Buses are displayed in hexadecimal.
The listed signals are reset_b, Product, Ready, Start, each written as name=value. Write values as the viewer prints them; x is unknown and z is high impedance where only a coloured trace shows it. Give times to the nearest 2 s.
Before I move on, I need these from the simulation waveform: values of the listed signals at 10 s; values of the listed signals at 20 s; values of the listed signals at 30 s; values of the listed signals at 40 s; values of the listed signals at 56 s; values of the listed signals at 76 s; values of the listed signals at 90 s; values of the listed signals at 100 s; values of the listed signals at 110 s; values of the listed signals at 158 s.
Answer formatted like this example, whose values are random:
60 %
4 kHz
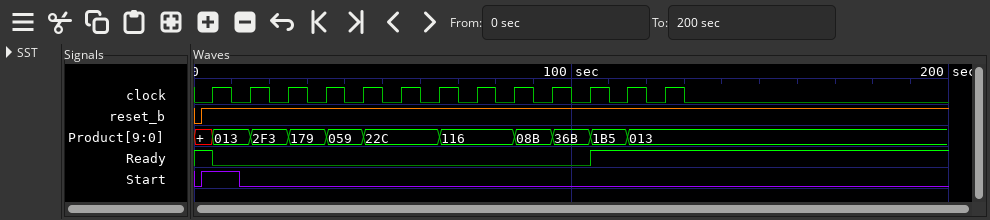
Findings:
reset_b=1, Product=013, Ready=0, Start=1
reset_b=1, Product=2F3, Ready=0, Start=0
reset_b=1, Product=179, Ready=0, Start=0
reset_b=1, Product=059, Ready=0, Start=0
reset_b=1, Product=22C, Ready=0, Start=0
reset_b=1, Product=116, Ready=0, Start=0
reset_b=1, Product=08B, Ready=0, Start=0
reset_b=1, Product=36B, Ready=0, Start=0
reset_b=1, Product=1B5, Ready=1, Start=0
reset_b=1, Product=013, Ready=1, Start=0
